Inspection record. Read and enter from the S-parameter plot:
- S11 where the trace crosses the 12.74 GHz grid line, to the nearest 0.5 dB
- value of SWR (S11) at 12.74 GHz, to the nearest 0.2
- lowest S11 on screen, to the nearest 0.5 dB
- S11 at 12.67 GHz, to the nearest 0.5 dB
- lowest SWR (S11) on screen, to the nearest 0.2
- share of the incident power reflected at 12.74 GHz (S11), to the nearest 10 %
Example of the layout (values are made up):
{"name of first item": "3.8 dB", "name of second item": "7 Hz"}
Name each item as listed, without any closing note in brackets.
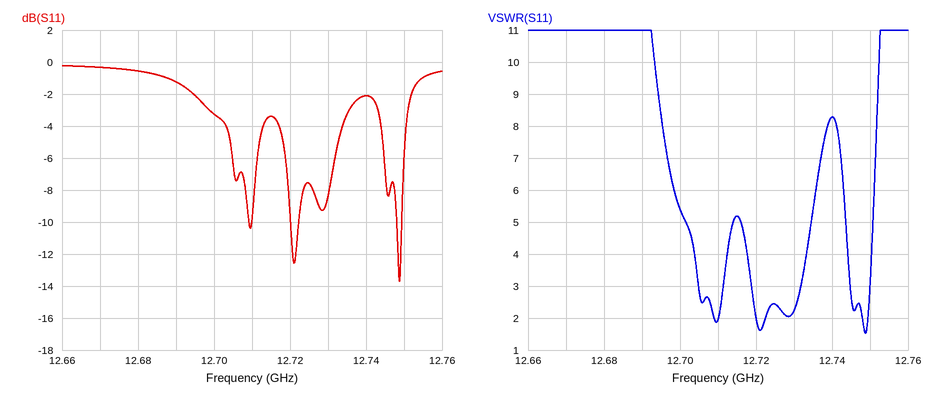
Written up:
{"S11 where the trace crosses the 12.74 GHz grid line, to the nearest 0.5 dB": "-2.0 dB", "value of SWR (S11) at 12.74 GHz, to the nearest 0.2": "8.2", "lowest S11 on screen, to the nearest 0.5 dB": "-13.5 dB", "S11 at 12.67 GHz, to the nearest 0.5 dB": "-0.5 dB", "lowest SWR (S11) on screen, to the nearest 0.2": "1.6", "share of the incident power reflected at 12.74 GHz (S11), to the nearest 10 %": "60 %"}
